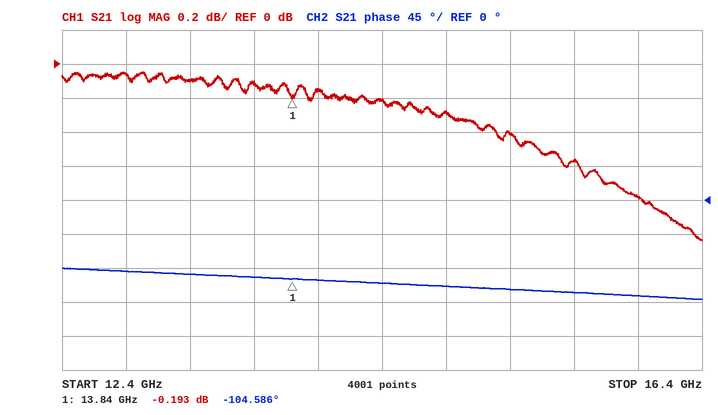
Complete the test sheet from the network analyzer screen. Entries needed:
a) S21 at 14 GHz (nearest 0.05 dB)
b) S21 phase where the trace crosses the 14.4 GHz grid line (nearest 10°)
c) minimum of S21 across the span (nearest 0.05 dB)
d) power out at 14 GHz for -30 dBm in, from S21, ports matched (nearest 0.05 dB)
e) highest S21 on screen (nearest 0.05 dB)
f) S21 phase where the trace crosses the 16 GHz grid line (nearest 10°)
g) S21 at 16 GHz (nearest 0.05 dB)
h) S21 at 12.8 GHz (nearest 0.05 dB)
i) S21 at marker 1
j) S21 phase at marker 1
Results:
-0.15 dB
-110°
-1.05 dB
-30.15 dBm
-0.05 dB
-130°
-0.80 dB
-0.05 dB
-0.193 dB
-104.586°
